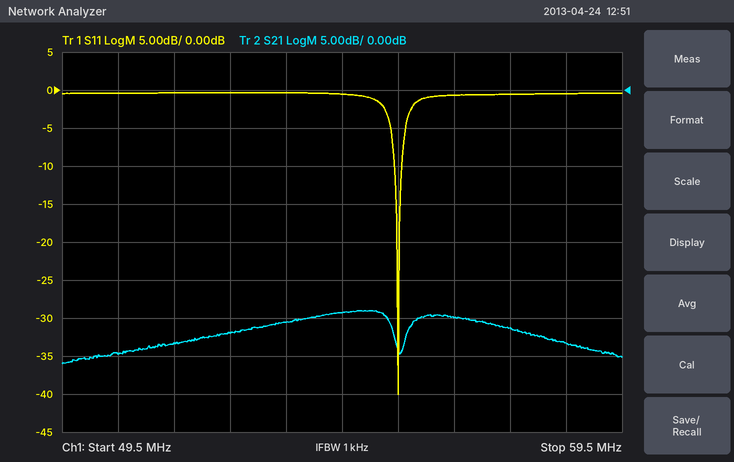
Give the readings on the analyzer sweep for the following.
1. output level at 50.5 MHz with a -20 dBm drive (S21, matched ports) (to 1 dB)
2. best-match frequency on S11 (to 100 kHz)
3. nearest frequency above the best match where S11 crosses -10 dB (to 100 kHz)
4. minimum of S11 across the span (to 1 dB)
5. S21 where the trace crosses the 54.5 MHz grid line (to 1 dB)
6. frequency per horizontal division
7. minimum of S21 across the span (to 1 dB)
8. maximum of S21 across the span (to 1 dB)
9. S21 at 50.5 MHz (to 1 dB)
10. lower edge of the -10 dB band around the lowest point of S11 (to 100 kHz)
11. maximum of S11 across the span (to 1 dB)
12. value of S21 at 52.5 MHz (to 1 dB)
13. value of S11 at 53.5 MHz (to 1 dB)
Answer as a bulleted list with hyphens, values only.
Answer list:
- -55 dBm
- 55.5 MHz
- 55.6 MHz
- -40 dB
- -29 dB
- 1 MHz
- -36 dB
- -29 dB
- -35 dB
- 55.4 MHz
- 0 dB
- -32 dB
- 0 dB
